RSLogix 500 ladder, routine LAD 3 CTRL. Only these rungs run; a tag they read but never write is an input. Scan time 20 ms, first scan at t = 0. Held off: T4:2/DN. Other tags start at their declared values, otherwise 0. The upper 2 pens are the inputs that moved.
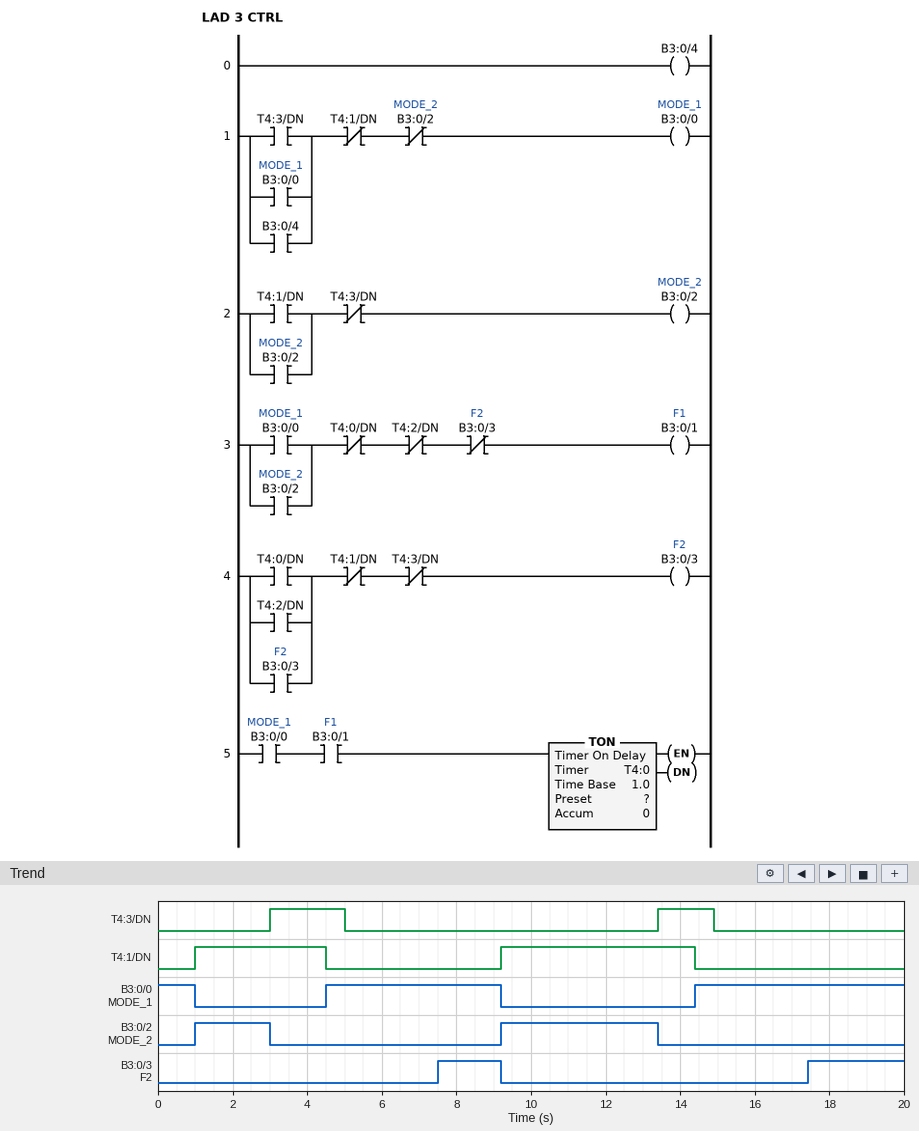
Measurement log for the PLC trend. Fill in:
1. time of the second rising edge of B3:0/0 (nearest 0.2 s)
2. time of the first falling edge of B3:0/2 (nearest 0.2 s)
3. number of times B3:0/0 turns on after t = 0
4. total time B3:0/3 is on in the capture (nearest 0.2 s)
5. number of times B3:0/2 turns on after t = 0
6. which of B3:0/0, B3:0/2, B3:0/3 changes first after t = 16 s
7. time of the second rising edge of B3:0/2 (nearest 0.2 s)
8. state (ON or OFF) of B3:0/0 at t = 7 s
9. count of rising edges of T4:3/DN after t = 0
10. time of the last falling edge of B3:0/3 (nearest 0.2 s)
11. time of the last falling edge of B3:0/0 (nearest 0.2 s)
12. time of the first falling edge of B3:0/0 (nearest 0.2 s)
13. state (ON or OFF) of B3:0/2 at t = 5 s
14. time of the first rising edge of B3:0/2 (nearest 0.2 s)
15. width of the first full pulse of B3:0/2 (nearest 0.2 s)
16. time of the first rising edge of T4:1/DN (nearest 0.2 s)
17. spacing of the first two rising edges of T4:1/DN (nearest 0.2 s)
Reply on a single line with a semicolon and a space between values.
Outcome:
14.4 s; 3.0 s; 2; 4.2 s; 2; B3:0/3; 9.2 s; ON; 2; 9.2 s; 9.2 s; 1.0 s; OFF; 1.0 s; 2.0 s; 1.0 s; 8.2 s
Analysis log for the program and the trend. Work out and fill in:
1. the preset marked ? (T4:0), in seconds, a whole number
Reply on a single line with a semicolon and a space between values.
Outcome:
3 s
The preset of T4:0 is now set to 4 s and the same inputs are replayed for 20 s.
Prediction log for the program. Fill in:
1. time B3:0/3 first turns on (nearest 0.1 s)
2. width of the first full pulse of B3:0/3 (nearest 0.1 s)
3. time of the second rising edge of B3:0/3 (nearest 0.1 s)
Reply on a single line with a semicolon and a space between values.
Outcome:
8.5 s; 0.7 s; 18.4 s
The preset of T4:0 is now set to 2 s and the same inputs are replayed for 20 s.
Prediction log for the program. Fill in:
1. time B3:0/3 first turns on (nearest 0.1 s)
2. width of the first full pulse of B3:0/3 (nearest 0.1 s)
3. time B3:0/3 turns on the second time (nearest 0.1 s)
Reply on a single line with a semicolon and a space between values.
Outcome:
6.5 s; 2.7 s; 16.4 s
